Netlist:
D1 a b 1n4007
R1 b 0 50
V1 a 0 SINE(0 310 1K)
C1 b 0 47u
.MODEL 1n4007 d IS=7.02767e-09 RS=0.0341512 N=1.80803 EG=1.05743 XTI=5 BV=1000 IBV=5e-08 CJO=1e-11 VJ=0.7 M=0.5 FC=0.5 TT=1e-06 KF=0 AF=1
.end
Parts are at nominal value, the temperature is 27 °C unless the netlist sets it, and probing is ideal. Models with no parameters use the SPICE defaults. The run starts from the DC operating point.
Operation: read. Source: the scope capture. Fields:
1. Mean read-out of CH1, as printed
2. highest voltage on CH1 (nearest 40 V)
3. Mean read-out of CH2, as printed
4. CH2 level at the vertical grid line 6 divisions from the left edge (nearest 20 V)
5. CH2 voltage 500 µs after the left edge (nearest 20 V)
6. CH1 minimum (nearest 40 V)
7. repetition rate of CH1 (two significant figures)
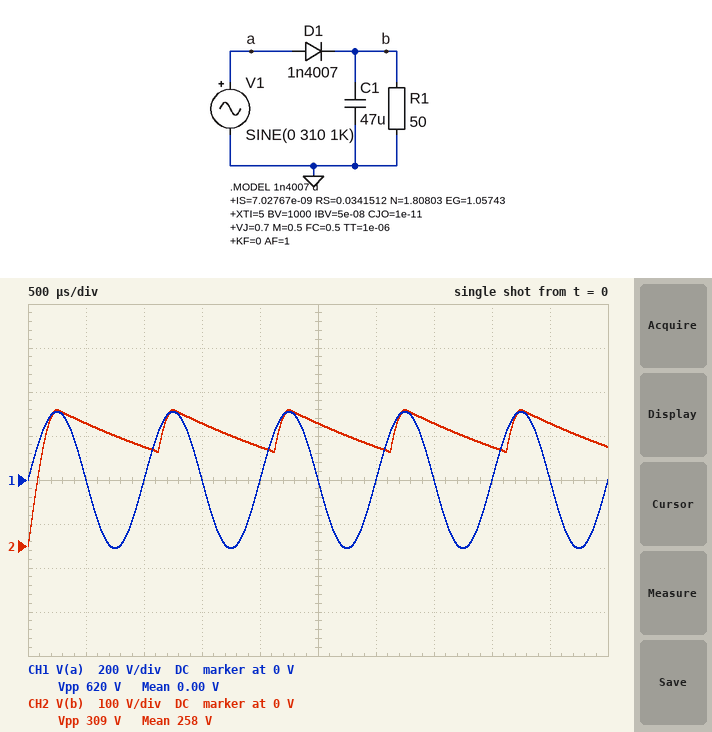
0.00 V
320 V
258 V
220 V
280 V
-320 V
1.0 kHz
